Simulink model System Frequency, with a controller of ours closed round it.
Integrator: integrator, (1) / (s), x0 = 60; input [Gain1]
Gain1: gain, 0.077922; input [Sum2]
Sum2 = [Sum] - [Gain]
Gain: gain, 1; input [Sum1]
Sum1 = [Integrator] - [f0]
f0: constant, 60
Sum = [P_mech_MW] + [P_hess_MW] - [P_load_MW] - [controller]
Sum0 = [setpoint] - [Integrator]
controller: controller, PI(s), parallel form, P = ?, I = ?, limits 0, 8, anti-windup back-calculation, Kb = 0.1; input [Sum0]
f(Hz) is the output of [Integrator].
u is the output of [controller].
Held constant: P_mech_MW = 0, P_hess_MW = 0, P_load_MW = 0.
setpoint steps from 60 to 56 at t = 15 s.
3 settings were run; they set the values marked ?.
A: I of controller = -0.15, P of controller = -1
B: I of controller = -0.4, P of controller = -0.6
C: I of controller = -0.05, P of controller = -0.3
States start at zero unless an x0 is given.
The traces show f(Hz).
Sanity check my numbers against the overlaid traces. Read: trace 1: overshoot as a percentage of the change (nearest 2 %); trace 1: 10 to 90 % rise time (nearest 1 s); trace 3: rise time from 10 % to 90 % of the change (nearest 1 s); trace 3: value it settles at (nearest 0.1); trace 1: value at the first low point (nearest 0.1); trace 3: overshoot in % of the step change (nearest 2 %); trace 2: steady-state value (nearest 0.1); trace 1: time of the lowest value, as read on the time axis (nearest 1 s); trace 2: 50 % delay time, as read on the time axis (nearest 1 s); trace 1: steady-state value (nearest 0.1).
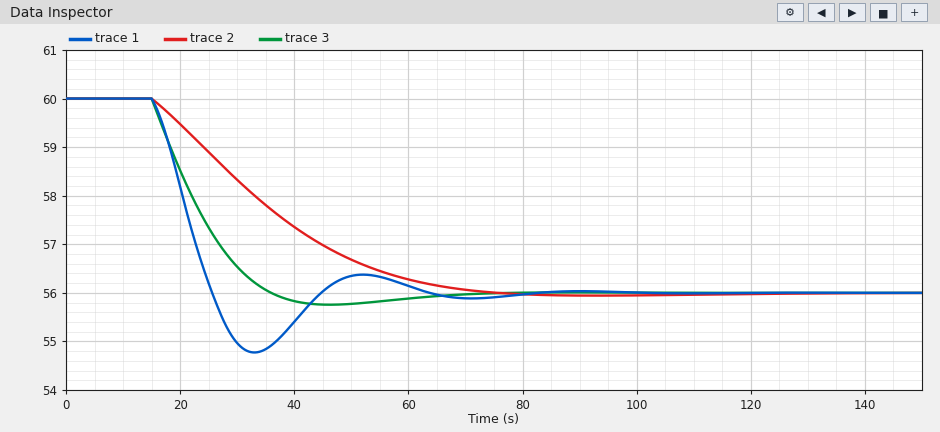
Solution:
30 %
8 s
15 s
56.0
54.8
6 %
56.0
33 s
33 s
56.0
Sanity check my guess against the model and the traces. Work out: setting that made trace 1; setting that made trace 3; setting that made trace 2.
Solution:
B
A
C
